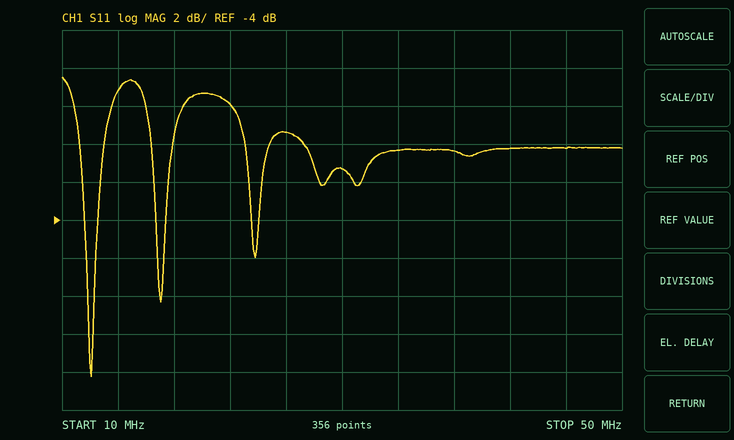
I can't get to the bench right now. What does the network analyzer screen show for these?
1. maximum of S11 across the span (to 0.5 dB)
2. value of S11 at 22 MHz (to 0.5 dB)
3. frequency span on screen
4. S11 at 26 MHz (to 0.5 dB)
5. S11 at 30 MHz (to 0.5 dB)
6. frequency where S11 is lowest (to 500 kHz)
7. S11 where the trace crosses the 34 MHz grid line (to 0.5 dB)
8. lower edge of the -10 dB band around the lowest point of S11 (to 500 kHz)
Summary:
3.5 dB
2.0 dB
40 MHz
0.5 dB
-1.5 dB
12.0 MHz
-0.5 dB
12.0 MHz
